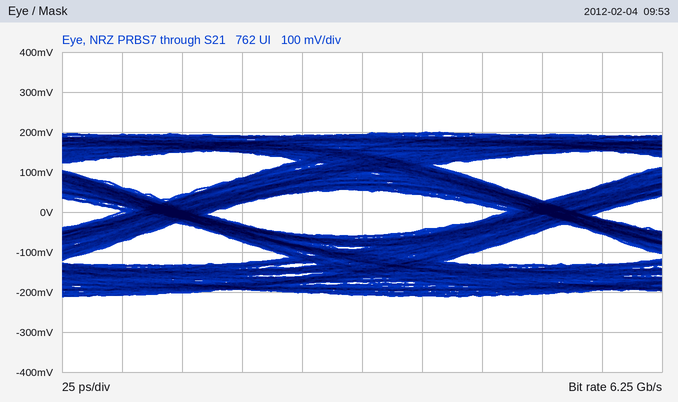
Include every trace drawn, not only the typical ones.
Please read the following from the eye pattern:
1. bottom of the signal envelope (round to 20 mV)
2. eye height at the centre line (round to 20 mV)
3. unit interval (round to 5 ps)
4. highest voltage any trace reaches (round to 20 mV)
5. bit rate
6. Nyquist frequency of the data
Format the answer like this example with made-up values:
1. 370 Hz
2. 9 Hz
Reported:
1. -220 mV
2. 120 mV
3. 160 ps
4. 200 mV
5. 6.25 Gb/s
6. 3.125 GHz
